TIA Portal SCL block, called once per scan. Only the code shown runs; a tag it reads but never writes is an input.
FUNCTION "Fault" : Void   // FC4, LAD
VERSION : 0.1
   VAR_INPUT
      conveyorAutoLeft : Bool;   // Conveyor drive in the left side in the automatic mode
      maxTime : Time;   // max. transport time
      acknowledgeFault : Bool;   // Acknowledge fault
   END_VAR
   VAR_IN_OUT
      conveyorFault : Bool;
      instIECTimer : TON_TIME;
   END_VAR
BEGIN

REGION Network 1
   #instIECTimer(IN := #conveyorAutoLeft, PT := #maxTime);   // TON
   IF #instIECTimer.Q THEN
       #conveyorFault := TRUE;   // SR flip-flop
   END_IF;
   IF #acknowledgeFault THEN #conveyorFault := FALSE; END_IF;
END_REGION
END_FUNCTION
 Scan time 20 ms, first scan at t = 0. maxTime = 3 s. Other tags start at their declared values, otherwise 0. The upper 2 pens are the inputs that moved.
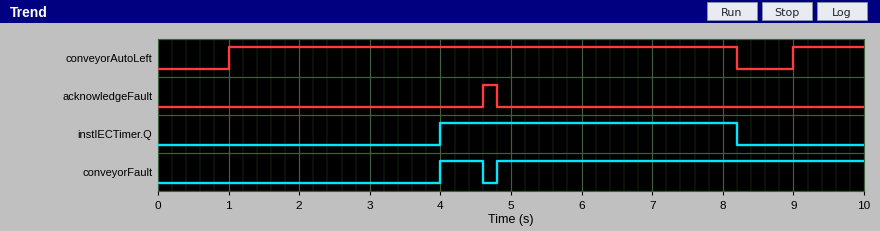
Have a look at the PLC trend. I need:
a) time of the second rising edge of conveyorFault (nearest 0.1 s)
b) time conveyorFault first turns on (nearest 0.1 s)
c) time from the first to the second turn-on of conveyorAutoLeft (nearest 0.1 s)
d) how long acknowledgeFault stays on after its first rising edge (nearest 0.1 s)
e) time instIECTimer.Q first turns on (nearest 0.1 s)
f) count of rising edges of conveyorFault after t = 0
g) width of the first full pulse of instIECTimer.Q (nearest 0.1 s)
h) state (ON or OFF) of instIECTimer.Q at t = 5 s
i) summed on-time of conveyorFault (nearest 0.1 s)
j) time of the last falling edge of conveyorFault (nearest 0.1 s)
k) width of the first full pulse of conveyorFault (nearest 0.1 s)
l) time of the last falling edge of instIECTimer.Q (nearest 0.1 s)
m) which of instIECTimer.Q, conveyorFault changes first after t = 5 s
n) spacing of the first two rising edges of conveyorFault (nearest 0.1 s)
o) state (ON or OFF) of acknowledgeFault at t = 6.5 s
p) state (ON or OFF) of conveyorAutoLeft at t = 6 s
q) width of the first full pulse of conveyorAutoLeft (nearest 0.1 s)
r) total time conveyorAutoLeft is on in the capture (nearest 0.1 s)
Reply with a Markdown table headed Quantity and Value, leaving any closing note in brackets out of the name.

| Quantity | Value |
|---|---|
| time of the second rising edge of conveyorFault | 4.8 s |
| time conveyorFault first turns on | 4.0 s |
| time from the first to the second turn-on of conveyorAutoLeft | 8.0 s |
| how long acknowledgeFault stays on after its first rising edge | 0.2 s |
| time instIECTimer.Q first turns on | 4.0 s |
| count of rising edges of conveyorFault after t = 0 | 2 |
| width of the first full pulse of instIECTimer.Q | 4.2 s |
| state (ON or OFF) of instIECTimer.Q at t = 5 s | ON |
| summed on-time of conveyorFault | 5.8 s |
| time of the last falling edge of conveyorFault | 4.6 s |
| width of the first full pulse of conveyorFault | 0.6 s |
| time of the last falling edge of instIECTimer.Q | 8.2 s |
| which of instIECTimer.Q, conveyorFault changes first after t = 5 s | instIECTimer.Q |
| spacing of the first two rising edges of conveyorFault | 0.8 s |
| state (ON or OFF) of acknowledgeFault at t = 6.5 s | OFF |
| state (ON or OFF) of conveyorAutoLeft at t = 6 s | ON |
| width of the first full pulse of conveyorAutoLeft | 7.2 s |
| total time conveyorAutoLeft is on in the capture | 8.2 s |
